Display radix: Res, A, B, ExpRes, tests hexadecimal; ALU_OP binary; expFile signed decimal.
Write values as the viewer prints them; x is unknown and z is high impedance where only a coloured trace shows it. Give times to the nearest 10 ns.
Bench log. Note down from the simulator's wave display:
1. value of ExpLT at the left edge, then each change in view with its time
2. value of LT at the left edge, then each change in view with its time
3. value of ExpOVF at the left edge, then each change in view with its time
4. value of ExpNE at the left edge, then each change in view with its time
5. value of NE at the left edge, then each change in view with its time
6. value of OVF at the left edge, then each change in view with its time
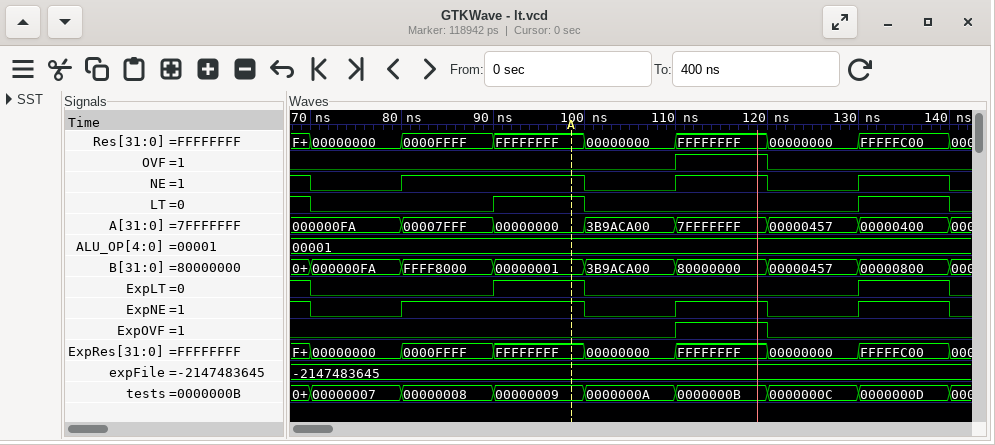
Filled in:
1, 0 at 70 ns, 1 at 90 ns, 0 at 100 ns, 1 at 130 ns, 0 at 140 ns
1, 0 at 70 ns, 1 at 90 ns, 0 at 100 ns, 1 at 130 ns, 0 at 140 ns
0, 1 at 110 ns, 0 at 120 ns
1, 0 at 70 ns, 1 at 80 ns, 0 at 100 ns, 1 at 110 ns, 0 at 120 ns, 1 at 130 ns, 0 at 140 ns
1, 0 at 70 ns, 1 at 80 ns, 0 at 100 ns, 1 at 110 ns, 0 at 120 ns, 1 at 130 ns, 0 at 140 ns
0, 1 at 110 ns, 0 at 120 ns
